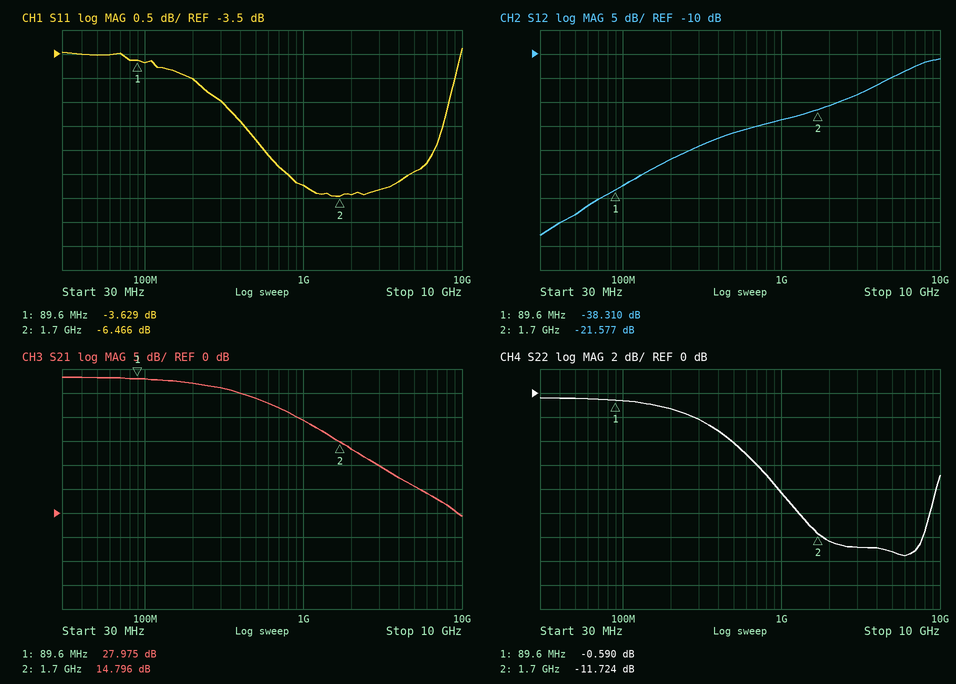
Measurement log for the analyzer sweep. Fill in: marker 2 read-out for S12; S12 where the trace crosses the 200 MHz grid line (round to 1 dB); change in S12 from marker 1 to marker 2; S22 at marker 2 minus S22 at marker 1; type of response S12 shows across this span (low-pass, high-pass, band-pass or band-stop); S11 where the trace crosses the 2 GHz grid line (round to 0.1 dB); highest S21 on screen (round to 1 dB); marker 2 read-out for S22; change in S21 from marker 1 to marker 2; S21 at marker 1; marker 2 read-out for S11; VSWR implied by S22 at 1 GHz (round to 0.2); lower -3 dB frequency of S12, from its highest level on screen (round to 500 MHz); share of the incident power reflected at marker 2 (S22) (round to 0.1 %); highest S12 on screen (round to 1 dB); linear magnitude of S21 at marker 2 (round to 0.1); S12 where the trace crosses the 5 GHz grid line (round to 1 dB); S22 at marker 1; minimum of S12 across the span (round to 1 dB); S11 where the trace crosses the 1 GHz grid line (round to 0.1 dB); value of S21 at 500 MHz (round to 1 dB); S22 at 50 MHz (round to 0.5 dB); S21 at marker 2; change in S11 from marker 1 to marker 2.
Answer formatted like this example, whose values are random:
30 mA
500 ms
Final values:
-21.577 dB
-32 dB
16.733 dB
-11.134 dB
high-pass
-6.4 dB
28 dB
-11.724 dB
-13.179 dB
27.975 dB
-6.466 dB
2.2
5.5 GHz
6.7 %
-11 dB
5.5
-15 dB
-0.590 dB
-48 dB
-6.2 dB
24 dB
-0.5 dB
14.796 dB
-2.837 dB
